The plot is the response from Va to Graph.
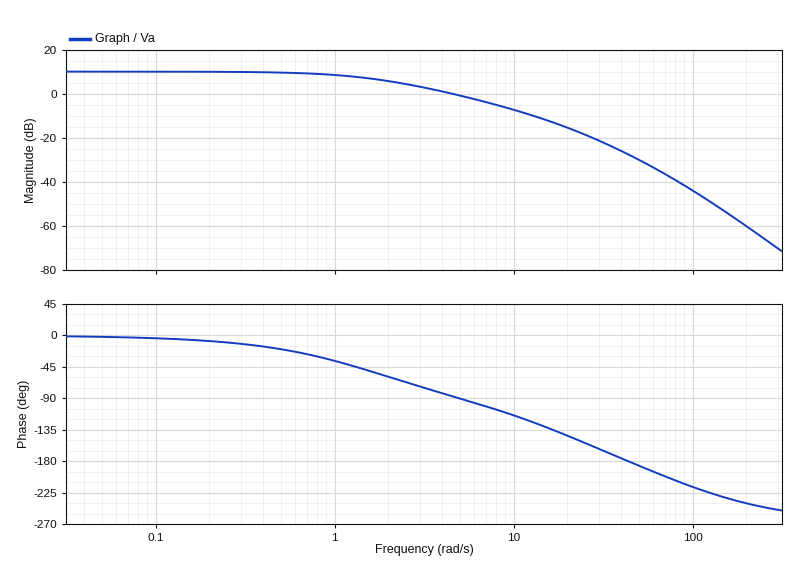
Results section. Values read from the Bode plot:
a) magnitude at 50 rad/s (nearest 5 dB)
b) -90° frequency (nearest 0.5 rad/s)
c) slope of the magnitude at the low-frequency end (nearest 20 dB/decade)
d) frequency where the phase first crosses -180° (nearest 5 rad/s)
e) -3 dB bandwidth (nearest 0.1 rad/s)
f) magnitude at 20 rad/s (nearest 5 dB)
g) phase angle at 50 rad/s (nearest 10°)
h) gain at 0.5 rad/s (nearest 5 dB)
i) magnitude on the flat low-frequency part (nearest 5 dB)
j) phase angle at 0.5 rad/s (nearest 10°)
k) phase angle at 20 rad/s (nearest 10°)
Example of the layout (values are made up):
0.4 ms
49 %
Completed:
-30 dB
5.0 rad/s
0 dB/decade
45 rad/s
1.5 rad/s
-15 dB
-190°
10 dB
10 dB
-20°
-140°
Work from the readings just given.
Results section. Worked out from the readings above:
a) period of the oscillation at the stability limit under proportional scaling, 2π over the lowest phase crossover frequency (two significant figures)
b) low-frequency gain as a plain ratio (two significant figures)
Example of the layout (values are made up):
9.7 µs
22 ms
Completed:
0.14 s
3.2
